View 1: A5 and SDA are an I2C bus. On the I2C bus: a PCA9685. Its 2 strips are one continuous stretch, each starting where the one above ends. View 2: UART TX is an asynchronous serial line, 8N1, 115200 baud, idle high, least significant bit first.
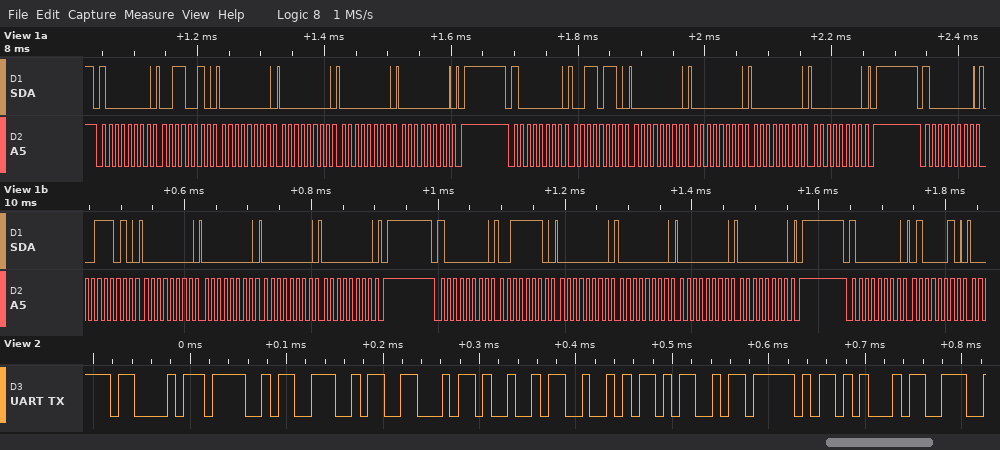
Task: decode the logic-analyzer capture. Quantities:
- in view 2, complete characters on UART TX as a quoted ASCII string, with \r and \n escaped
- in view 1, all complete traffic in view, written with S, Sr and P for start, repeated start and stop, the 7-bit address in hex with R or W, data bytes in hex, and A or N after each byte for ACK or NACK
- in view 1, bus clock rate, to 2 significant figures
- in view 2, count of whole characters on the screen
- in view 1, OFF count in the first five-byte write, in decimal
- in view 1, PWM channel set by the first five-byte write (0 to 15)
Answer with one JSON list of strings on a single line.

["\"CONFIRM_E\"", "S 40W A 32 A 00 A 00 A 00 A 00 A P S 40W A 36 A 00 A 00 A 00 A 00 A P S 40W A 3A A 00 A 00 A 00 A 00 A P S 40W A 3E A 00 A 00 A 00 A 00 A P S 40W A 42 A", "100 kHz", "9", "0", "11"]
